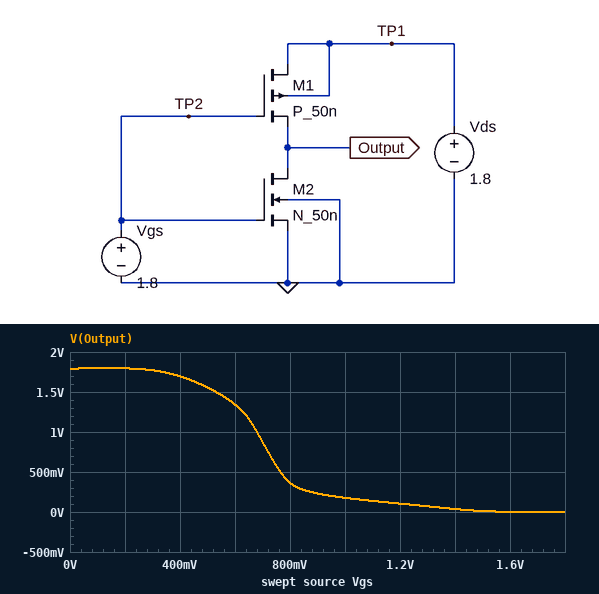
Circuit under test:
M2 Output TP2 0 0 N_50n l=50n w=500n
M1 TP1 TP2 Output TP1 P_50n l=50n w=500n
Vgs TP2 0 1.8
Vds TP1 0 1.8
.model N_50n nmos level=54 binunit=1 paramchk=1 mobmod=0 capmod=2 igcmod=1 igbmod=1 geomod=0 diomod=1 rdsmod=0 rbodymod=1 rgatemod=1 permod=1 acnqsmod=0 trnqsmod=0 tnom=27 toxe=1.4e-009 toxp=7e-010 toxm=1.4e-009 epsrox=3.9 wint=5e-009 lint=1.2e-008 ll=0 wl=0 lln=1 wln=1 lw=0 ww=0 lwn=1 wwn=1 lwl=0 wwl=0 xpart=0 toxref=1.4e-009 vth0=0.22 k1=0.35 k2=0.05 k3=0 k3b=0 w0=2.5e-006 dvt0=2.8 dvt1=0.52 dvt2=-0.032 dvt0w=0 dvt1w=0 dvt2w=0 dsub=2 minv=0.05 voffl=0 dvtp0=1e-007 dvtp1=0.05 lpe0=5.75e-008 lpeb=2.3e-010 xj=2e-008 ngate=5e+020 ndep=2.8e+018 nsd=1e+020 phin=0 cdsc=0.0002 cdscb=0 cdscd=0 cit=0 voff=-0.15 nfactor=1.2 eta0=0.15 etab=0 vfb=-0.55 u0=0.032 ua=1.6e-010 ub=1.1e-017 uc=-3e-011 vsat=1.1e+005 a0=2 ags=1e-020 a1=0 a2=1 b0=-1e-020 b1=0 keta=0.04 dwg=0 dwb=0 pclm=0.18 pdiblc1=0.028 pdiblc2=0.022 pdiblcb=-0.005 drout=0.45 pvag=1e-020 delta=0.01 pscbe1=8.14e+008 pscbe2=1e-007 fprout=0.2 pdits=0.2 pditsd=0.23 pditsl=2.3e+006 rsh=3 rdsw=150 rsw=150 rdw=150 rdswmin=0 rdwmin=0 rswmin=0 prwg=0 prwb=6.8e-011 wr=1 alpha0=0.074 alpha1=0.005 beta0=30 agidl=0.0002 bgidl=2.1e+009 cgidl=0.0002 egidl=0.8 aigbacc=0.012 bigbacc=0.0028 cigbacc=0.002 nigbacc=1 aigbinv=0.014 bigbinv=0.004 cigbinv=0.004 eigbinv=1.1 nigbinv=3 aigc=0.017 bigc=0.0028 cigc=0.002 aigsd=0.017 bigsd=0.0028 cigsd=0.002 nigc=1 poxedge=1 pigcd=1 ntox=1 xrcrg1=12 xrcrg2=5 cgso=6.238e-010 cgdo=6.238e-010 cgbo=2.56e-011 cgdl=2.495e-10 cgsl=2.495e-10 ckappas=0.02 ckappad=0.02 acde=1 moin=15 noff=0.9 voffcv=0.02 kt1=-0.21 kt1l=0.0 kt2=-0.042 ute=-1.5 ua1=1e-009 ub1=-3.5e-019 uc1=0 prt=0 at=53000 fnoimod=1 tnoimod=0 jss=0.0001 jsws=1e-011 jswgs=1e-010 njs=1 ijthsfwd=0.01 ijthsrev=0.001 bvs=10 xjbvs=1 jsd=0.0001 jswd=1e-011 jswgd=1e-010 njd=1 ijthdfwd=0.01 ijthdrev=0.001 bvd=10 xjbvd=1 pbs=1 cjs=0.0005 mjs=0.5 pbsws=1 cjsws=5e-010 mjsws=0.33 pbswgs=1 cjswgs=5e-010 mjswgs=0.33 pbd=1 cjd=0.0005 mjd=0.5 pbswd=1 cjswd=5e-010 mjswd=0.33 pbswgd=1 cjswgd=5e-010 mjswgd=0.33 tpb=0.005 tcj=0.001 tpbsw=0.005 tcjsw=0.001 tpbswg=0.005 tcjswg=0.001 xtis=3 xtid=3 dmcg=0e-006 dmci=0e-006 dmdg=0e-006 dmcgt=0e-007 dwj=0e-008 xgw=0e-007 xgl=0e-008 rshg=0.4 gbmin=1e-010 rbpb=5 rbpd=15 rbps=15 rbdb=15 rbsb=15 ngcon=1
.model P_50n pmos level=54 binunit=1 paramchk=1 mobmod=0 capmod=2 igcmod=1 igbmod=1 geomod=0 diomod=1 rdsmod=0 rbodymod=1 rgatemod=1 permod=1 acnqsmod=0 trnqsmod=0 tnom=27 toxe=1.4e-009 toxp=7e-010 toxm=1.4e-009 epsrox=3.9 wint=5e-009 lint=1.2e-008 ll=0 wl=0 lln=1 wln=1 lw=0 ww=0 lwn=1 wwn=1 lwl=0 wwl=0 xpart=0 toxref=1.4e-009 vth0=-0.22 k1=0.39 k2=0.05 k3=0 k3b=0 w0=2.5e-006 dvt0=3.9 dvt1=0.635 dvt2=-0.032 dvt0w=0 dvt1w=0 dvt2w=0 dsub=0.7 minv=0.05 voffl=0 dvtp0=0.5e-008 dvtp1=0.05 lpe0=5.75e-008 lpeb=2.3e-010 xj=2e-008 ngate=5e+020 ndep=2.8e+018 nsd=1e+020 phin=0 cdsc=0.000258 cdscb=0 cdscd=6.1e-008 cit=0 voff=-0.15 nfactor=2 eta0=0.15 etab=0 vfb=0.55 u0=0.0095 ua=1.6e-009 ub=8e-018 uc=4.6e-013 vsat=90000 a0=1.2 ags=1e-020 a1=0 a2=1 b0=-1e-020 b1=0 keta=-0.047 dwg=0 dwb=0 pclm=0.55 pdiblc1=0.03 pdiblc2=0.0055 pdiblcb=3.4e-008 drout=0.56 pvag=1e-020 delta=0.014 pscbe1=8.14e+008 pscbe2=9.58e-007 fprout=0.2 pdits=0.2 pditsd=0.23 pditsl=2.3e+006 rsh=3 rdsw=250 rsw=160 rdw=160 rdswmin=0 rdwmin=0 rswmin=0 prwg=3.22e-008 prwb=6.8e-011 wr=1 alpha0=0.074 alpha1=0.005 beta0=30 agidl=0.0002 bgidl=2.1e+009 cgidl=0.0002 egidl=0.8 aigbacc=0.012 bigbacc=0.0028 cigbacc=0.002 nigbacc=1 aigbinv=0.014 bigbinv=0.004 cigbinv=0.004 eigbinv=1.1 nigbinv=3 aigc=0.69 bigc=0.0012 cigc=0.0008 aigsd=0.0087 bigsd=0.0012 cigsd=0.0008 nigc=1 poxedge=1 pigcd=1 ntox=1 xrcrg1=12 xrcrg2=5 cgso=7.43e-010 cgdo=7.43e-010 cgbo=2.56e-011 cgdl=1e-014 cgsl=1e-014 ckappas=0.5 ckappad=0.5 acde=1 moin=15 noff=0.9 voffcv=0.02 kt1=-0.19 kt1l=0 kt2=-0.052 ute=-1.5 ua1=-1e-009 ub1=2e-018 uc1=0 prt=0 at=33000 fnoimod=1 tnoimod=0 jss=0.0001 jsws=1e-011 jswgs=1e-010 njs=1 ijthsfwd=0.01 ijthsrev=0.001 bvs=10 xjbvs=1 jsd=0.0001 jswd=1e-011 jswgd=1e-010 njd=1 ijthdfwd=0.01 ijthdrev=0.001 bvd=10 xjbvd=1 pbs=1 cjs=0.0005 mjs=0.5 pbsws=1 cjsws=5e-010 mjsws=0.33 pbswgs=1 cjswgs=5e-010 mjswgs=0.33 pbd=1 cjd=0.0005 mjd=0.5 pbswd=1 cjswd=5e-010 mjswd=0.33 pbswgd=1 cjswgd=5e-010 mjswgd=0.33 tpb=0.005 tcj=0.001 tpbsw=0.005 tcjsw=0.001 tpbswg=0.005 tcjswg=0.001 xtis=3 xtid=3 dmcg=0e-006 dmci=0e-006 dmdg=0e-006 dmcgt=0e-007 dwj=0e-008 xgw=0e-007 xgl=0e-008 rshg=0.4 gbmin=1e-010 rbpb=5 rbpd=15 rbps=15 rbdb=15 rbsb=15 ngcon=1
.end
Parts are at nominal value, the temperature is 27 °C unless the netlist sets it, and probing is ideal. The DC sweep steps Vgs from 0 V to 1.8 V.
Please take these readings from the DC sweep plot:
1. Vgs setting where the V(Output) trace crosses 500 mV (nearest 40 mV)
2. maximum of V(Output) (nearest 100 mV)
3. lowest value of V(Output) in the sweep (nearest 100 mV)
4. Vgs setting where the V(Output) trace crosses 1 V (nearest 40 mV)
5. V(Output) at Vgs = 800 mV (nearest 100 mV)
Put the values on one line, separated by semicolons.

760 mV; 1.8 V; 0 V; 680 mV; 400 mV
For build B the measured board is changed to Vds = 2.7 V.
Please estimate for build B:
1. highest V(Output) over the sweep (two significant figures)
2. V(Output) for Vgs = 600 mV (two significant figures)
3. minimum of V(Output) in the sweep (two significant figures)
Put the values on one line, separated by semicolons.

2.4 V; 2.0 V; 460 mV
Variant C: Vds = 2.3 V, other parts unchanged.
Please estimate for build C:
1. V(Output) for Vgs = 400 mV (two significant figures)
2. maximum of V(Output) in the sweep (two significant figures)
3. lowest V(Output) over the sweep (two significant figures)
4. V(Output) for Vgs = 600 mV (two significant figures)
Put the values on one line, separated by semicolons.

2.0 V; 2.2 V; 190 mV; 1.8 V
